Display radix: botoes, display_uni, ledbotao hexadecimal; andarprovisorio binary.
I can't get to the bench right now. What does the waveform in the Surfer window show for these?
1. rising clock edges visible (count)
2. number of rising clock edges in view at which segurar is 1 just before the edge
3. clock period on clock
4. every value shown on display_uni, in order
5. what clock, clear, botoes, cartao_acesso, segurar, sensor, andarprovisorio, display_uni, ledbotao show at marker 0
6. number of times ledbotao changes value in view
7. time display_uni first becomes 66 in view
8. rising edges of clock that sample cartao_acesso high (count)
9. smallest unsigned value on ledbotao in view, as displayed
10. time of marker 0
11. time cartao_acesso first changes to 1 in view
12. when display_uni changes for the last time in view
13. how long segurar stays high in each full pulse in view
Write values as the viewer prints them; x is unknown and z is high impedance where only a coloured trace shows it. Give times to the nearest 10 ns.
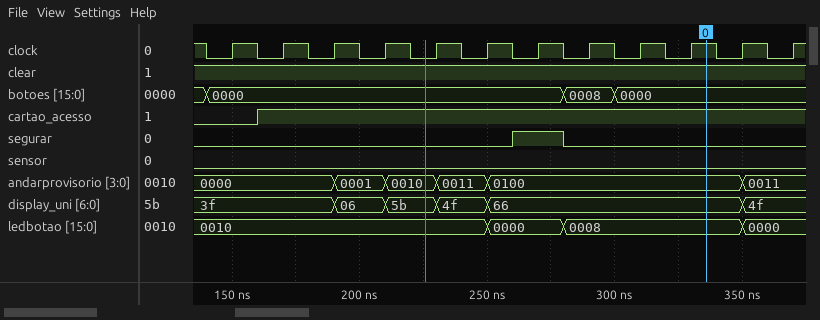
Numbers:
12
1
20 ns
3f, 06, 5b, 4f, 66, 4f
clock=1, clear=1, botoes=0000, cartao_acesso=1, segurar=0, sensor=0, andarprovisorio=0100, display_uni=66, ledbotao=0008
3
250 ns
11
0000
340 ns
160 ns
350 ns
20 ns
